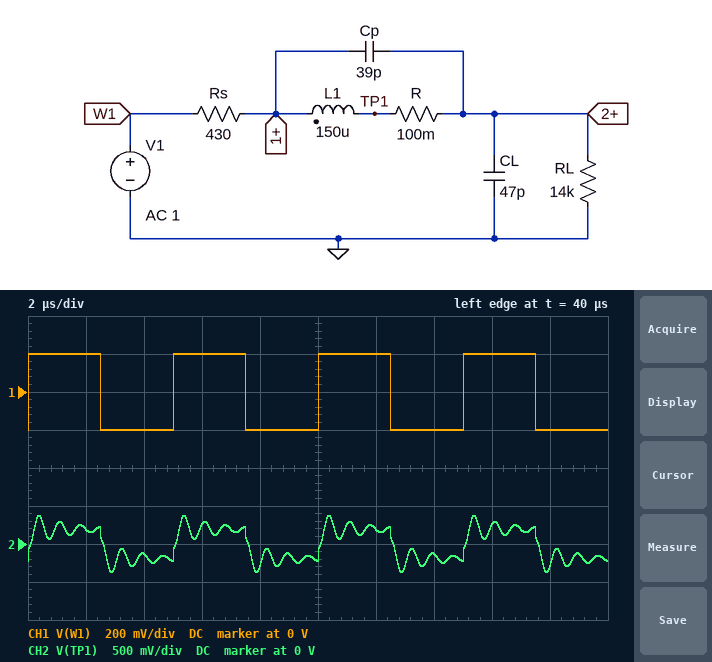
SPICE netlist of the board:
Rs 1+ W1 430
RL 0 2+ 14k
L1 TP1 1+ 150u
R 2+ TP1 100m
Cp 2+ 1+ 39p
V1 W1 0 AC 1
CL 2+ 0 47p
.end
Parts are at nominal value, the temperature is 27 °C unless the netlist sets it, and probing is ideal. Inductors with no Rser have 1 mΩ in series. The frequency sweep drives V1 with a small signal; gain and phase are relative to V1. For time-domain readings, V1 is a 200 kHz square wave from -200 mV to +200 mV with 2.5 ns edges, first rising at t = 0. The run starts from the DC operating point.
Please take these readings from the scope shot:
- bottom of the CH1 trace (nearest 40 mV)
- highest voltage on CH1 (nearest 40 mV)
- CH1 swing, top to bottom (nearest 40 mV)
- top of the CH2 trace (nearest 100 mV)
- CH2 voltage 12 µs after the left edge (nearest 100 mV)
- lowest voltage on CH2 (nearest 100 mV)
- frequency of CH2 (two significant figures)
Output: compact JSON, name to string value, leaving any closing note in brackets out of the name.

{"bottom of the CH1 trace": "-200 mV", "highest voltage on CH1": "200 mV", "CH1 swing, top to bottom": "400 mV", "top of the CH2 trace": "400 mV", "CH2 voltage 12 µs after the left edge": "200 mV", "lowest voltage on CH2": "-400 mV", "frequency of CH2": "200 kHz"}
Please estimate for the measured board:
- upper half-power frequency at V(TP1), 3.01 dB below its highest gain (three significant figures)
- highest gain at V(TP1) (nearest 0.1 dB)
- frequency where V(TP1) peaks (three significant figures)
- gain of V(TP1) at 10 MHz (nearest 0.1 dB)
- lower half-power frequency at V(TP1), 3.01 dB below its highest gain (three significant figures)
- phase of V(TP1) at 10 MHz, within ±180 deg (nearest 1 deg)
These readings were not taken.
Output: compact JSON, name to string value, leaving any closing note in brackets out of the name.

{"upper half-power frequency at V(TP1), 3.01 dB below its highest gain": "1.50 MHz", "highest gain at V(TP1)": "9.1 dB", "frequency where V(TP1) peaks": "1.39 MHz", "gain of V(TP1) at 10 MHz": "-8.3 dB", "lower half-power frequency at V(TP1), 3.01 dB below its highest gain": "1.21 MHz", "phase of V(TP1) at 10 MHz, within ±180 deg": "-28 deg"}
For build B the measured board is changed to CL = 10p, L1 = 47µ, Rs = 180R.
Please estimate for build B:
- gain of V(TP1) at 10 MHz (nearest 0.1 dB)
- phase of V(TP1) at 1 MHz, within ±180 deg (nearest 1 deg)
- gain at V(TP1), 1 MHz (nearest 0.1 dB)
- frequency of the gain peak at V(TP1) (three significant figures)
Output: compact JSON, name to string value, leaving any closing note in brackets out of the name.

{"gain of V(TP1) at 10 MHz": "-2.4 dB", "phase of V(TP1) at 1 MHz, within ±180 deg": "-2 deg", "gain at V(TP1), 1 MHz": "0.1 dB", "frequency of the gain peak at V(TP1)": "3.28 MHz"}
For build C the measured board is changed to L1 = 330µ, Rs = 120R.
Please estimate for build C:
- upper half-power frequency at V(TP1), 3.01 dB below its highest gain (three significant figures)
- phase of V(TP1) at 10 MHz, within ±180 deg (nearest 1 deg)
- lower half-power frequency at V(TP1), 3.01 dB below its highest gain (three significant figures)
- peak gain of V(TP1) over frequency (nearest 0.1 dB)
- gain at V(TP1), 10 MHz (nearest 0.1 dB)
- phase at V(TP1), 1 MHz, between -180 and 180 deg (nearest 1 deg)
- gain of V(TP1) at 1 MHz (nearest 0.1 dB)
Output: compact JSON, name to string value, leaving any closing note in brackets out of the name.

{"upper half-power frequency at V(TP1), 3.01 dB below its highest gain": "998 kHz", "phase of V(TP1) at 10 MHz, within ±180 deg": "-8 deg", "lower half-power frequency at V(TP1), 3.01 dB below its highest gain": "839 kHz", "peak gain of V(TP1) over frequency": "10.9 dB", "gain at V(TP1), 10 MHz": "-7.1 dB", "phase at V(TP1), 1 MHz, between -180 and 180 deg": "-125 deg", "gain of V(TP1) at 1 MHz": "7.7 dB"}
